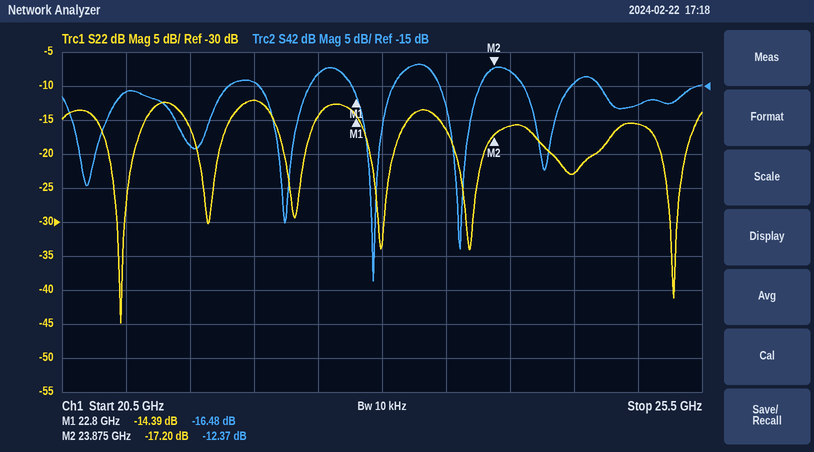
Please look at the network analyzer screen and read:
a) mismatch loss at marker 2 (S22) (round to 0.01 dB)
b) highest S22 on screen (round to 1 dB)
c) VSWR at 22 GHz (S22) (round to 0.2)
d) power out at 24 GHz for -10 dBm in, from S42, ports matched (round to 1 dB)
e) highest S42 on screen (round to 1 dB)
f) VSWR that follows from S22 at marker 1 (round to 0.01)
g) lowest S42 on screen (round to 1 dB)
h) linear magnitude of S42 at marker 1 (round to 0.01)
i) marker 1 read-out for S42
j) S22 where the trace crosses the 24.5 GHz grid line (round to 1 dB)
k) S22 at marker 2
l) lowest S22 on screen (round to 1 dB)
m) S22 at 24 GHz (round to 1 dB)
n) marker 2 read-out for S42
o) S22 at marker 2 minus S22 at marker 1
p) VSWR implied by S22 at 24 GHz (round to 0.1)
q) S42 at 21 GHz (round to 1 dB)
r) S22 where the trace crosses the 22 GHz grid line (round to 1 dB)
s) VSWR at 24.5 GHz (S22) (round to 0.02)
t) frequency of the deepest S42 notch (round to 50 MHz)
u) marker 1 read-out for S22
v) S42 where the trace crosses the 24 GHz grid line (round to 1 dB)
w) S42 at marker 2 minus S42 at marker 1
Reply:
0.08 dB
-12 dB
1.6
-23 dBm
-12 dB
1.47
-44 dB
0.15
-16.48 dB
-23 dB
-17.20 dB
-45 dB
-16 dB
-12.37 dB
-2.81 dB
1.4
-16 dB
-12 dB
1.16
22.95 GHz
-14.39 dB
-13 dB
4.11 dB
